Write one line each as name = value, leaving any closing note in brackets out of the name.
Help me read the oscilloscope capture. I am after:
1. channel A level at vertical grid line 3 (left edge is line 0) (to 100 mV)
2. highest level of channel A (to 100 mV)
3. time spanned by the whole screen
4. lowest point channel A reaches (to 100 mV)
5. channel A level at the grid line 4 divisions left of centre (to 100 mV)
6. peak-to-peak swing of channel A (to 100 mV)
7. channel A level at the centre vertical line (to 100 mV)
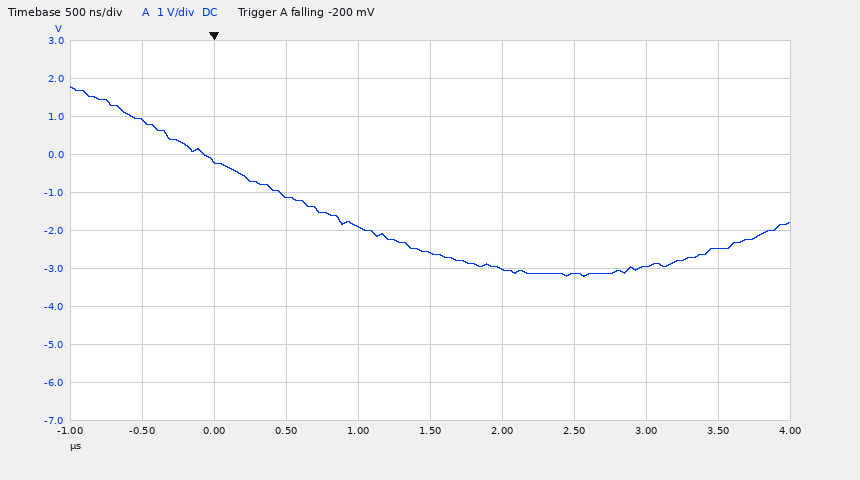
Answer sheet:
channel A level at vertical grid line 3 (left edge is line 0) = -1.1 V
highest level of channel A = 1.8 V
time spanned by the whole screen = 5 µs
lowest point channel A reaches = -3.2 V
channel A level at the grid line 4 divisions left of centre = 900 mV
peak-to-peak swing of channel A = 5.0 V
channel A level at the centre vertical line = -2.6 V
